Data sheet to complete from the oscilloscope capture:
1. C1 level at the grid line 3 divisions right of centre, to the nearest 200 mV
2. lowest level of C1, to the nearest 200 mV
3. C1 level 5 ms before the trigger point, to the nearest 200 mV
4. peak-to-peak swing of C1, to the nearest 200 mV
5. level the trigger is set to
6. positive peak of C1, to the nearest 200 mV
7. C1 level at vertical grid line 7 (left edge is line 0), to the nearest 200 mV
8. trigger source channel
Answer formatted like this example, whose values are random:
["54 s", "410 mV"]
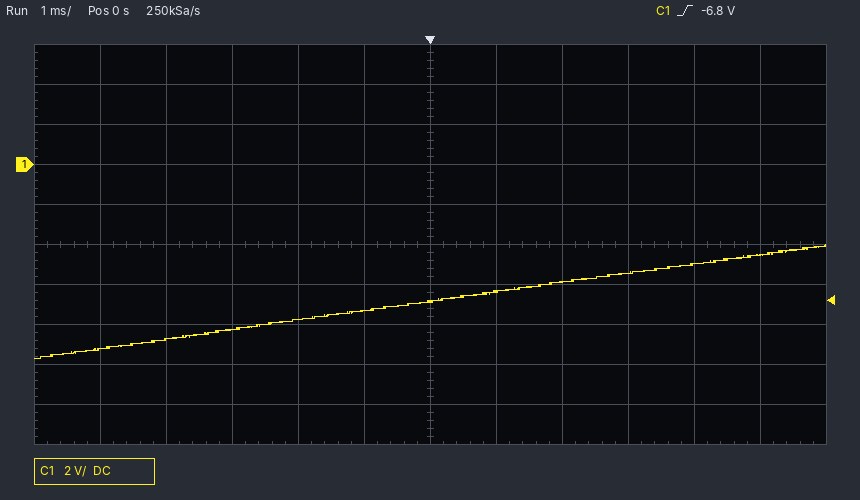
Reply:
["-5.4 V", "-9.6 V", "-9.2 V", "5.6 V", "-6.8 V", "-4.0 V", "-6.4 V", "C1"]
